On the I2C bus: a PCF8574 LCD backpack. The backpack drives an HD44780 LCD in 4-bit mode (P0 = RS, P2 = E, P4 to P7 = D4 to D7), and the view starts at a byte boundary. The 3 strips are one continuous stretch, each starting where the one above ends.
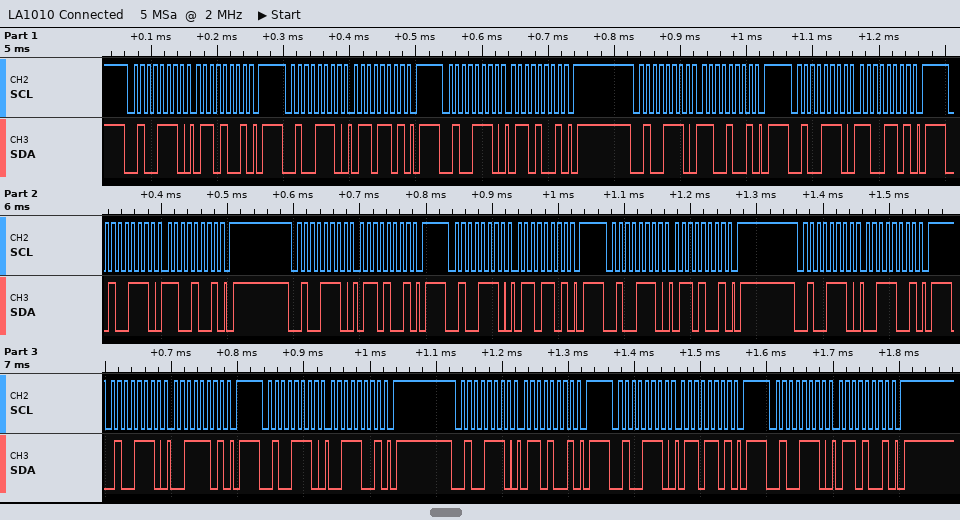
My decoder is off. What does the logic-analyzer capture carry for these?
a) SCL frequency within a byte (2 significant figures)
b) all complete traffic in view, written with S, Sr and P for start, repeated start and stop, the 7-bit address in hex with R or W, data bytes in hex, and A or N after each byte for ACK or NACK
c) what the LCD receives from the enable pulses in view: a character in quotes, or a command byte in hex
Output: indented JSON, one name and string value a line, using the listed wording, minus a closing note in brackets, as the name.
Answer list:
{
  "SCL frequency within a byte": "100 kHz",
  "all complete traffic in view, written with S, Sr and P for start, repeated start and stop, the 7-bit address in hex with R or W, data bytes in hex, and A or N after each byte for ACK or NACK": "S 27W A 69 A P S 27W A 6D A P S 27W A 69 A P S 27W A C9 A P S 27W A CD A P S 27W A C9 A P S 27W A 69 A P S 27W A 6D A P S 27W A 69 A P S 27W A 39 A P S 27W A 3D A P S 27W A 39 A P S 27W A 69 A P S 27W A 6D A P S 27W A 69 A P",
  "what the LCD receives from the enable pulses in view: a character in quotes, or a command byte in hex": "'l' 'c'"
}
